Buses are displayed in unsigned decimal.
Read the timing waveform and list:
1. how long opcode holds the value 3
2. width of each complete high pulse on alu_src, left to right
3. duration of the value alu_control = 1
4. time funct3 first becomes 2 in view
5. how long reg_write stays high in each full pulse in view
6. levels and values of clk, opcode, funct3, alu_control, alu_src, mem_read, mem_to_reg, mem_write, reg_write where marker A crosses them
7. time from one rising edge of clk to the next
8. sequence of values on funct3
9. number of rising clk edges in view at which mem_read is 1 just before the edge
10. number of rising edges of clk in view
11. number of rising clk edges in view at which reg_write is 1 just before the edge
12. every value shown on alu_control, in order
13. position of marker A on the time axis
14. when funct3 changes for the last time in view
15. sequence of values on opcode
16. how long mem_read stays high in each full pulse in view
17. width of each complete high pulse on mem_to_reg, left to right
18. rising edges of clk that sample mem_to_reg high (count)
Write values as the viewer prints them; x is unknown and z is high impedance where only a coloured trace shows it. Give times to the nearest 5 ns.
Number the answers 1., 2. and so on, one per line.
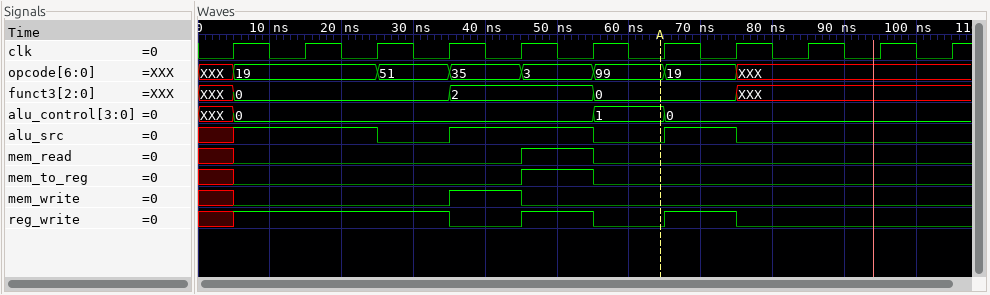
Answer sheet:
1. 10 ns
2. 20 ns, 10 ns
3. 10 ns
4. 35 ns
5. 10 ns, 10 ns
6. clk=0, opcode=99, funct3=0, alu_control=1, alu_src=0, mem_read=0, mem_to_reg=0, mem_write=0, reg_write=0
7. 10 ns
8. XXX, 0, 2, 0, XXX
9. 1
10. 11
11. 5
12. XXX, 0, 1, 0
13. 65 ns
14. 75 ns
15. XXX, 19, 51, 35, 3, 99, 19, XXX
16. 10 ns
17. 10 ns
18. 1
